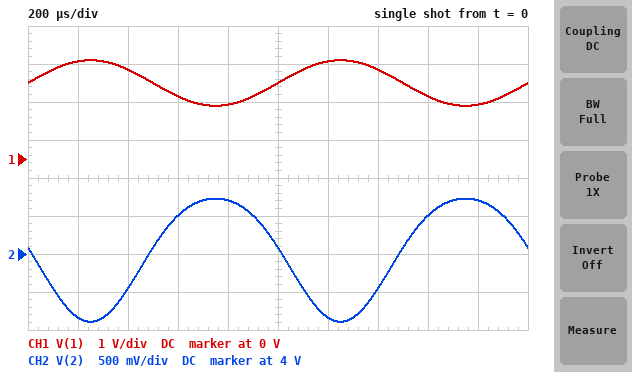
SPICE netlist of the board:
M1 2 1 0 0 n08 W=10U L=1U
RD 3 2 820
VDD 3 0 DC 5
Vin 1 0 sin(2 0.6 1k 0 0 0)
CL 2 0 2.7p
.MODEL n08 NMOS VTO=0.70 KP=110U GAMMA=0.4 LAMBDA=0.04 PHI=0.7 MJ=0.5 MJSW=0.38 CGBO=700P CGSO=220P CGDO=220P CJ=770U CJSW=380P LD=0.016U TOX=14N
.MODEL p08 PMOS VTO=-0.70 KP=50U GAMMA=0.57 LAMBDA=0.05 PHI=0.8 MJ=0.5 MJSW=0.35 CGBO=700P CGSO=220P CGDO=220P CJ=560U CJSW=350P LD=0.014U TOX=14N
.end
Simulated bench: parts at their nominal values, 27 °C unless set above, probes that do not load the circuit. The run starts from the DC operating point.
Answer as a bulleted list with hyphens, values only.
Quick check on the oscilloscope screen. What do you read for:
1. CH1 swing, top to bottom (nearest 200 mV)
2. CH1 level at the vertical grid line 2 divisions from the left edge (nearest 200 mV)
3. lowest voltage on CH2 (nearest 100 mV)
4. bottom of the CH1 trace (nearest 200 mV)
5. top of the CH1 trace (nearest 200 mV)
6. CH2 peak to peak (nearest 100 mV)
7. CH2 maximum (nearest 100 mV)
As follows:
- 1.2 V
- 2.4 V
- 3.1 V
- 1.4 V
- 2.6 V
- 1.6 V
- 4.7 V
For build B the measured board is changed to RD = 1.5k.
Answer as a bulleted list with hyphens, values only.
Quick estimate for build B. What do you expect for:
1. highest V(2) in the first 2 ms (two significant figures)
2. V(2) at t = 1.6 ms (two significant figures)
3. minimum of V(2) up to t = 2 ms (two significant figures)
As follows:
- 4.5 V
- 4.1 V
- 1.7 V
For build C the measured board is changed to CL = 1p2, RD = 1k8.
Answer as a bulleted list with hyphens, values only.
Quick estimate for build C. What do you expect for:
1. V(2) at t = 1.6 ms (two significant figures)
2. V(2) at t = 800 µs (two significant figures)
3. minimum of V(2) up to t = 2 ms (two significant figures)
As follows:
- 3.9 V
- 4.4 V
- 1.4 V
